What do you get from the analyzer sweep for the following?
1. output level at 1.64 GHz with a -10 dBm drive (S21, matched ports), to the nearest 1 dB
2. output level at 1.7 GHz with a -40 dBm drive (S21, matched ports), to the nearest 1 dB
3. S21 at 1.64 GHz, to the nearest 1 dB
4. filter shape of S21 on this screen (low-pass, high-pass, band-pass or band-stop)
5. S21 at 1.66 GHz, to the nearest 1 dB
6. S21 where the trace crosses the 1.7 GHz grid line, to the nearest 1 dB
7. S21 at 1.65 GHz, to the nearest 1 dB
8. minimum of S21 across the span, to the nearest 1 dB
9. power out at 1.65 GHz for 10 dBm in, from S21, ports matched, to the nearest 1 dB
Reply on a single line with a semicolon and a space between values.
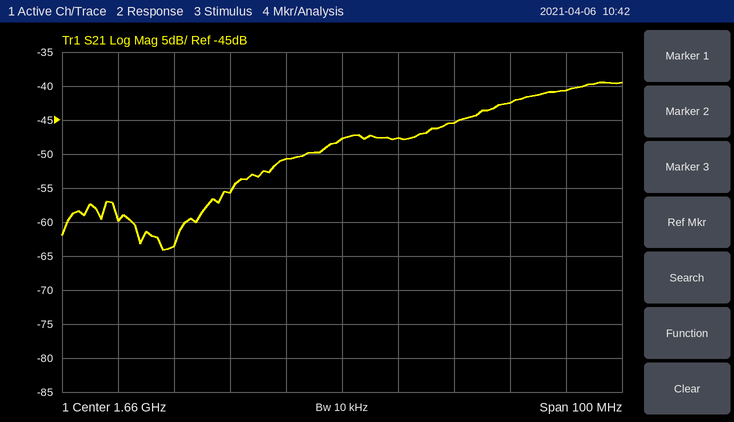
-66 dBm; -81 dBm; -56 dB; high-pass; -48 dB; -41 dB; -51 dB; -64 dB; -41 dBm
